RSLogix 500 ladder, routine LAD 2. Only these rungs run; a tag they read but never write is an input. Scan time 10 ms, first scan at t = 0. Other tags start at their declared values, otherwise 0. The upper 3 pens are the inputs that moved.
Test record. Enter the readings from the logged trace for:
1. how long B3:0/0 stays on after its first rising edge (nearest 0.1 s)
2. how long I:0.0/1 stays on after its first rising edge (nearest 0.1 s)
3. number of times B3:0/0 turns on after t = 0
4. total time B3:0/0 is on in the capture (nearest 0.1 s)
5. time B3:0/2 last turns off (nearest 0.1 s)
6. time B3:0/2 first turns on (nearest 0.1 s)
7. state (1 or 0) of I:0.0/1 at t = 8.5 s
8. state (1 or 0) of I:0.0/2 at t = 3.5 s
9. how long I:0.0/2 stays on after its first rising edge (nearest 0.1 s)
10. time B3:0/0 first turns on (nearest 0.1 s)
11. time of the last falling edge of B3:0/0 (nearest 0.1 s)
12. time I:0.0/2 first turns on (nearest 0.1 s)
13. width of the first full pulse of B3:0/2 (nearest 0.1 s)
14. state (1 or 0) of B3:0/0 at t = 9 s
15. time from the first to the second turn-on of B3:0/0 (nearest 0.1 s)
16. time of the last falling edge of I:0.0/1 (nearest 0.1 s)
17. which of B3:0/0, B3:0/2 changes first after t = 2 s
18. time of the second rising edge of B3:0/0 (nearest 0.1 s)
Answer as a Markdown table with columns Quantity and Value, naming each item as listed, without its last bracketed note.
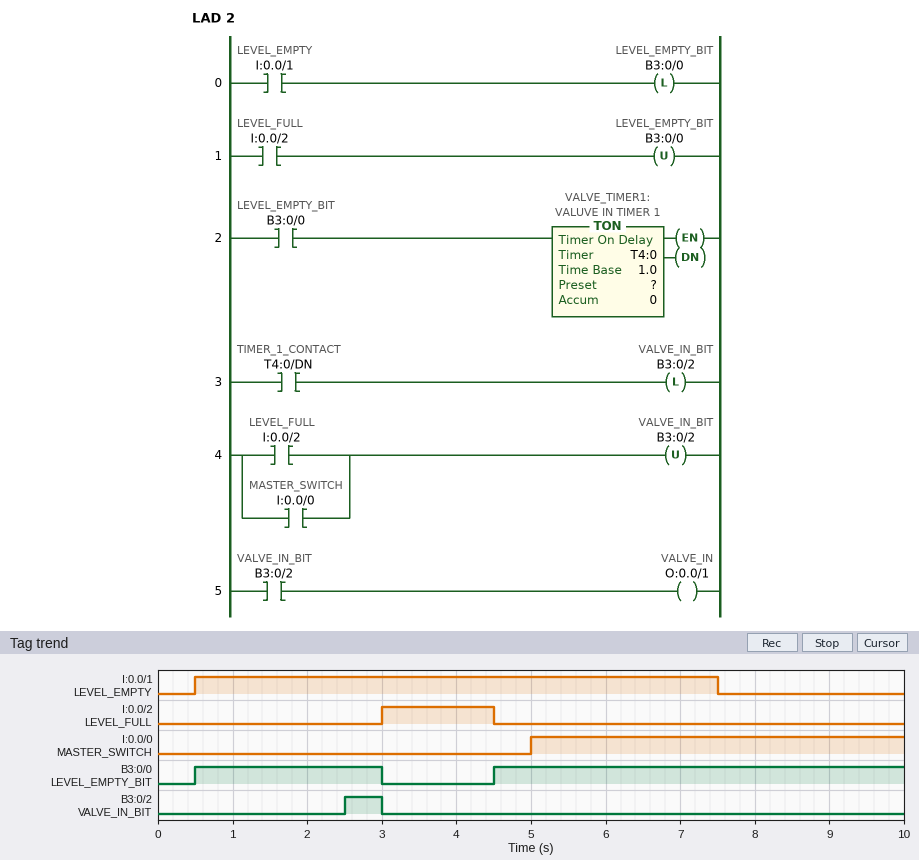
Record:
| Quantity | Value |
|---|---|
| how long B3:0/0 stays on after its first rising edge | 2.5 s |
| how long I:0.0/1 stays on after its first rising edge | 7.0 s |
| number of times B3:0/0 turns on after t = 0 | 2 |
| total time B3:0/0 is on in the capture | 8.0 s |
| time B3:0/2 last turns off | 3.0 s |
| time B3:0/2 first turns on | 2.5 s |
| state (1 or 0) of I:0.0/1 at t = 8.5 s | 0 |
| state (1 or 0) of I:0.0/2 at t = 3.5 s | 1 |
| how long I:0.0/2 stays on after its first rising edge | 1.5 s |
| time B3:0/0 first turns on | 0.5 s |
| time of the last falling edge of B3:0/0 | 3.0 s |
| time I:0.0/2 first turns on | 3.0 s |
| width of the first full pulse of B3:0/2 | 0.5 s |
| state (1 or 0) of B3:0/0 at t = 9 s | 1 |
| time from the first to the second turn-on of B3:0/0 | 4.0 s |
| time of the last falling edge of I:0.0/1 | 7.5 s |
| which of B3:0/0, B3:0/2 changes first after t = 2 s | B3:0/2 |
| time of the second rising edge of B3:0/0 | 4.5 s |
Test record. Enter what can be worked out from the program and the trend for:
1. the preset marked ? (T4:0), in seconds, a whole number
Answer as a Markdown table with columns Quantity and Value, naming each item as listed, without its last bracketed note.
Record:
| Quantity | Value |
|---|---|
| the preset marked ? (T4:0), in seconds, a whole number | 2 s |
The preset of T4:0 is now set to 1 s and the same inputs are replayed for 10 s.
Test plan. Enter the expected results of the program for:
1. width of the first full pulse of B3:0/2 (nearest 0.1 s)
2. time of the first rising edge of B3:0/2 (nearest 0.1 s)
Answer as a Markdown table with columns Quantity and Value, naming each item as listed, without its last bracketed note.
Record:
| Quantity | Value |
|---|---|
| width of the first full pulse of B3:0/2 | 1.5 s |
| time of the first rising edge of B3:0/2 | 1.5 s |
